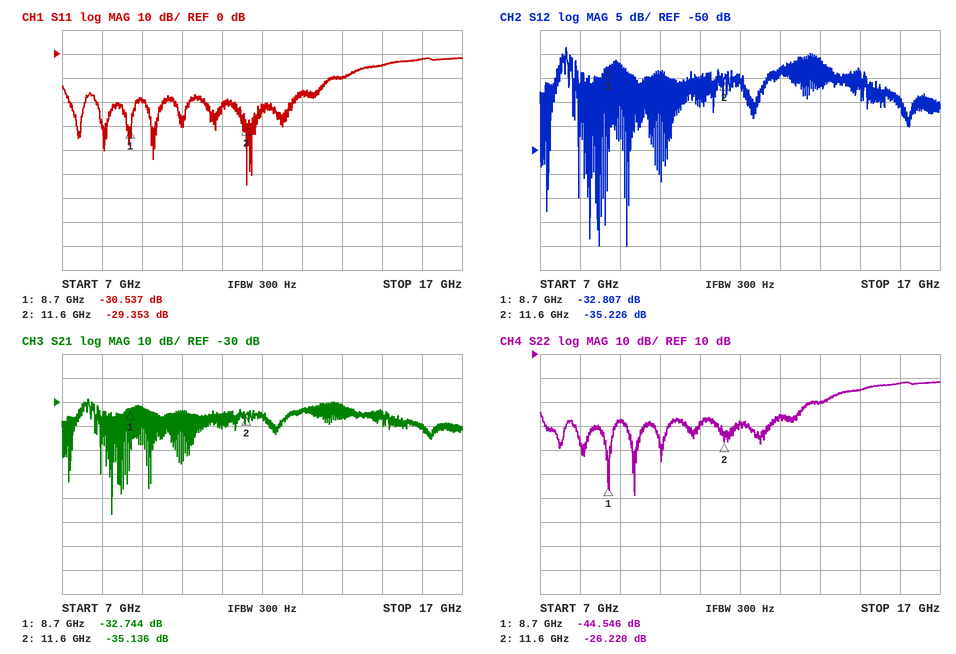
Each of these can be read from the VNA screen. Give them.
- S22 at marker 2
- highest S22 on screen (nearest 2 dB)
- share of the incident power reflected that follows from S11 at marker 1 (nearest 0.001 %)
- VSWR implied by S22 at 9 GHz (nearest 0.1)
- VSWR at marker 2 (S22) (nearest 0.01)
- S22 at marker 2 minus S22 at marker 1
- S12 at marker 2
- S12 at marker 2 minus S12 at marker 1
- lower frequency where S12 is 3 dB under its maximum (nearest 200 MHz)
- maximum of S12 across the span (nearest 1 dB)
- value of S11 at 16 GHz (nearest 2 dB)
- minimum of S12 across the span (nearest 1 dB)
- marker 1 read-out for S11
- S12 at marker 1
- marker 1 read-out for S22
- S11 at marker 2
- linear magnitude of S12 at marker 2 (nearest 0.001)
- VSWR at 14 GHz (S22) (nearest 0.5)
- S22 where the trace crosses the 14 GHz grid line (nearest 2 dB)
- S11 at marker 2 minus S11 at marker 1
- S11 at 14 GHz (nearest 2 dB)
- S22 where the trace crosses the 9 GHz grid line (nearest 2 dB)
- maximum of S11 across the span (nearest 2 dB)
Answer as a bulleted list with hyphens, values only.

- -26.220 dB
- -2 dB
- 0.088 %
- 1.3
- 1.10
- 18.326 dB
- -35.226 dB
- -2.419 dB
- 7.6 GHz
- -29 dB
- -2 dB
- -70 dB
- -30.537 dB
- -32.807 dB
- -44.546 dB
- -29.353 dB
- 0.017
- 2.0
- -10 dB
- 1.184 dB
- -10 dB
- -18 dB
- -2 dB
